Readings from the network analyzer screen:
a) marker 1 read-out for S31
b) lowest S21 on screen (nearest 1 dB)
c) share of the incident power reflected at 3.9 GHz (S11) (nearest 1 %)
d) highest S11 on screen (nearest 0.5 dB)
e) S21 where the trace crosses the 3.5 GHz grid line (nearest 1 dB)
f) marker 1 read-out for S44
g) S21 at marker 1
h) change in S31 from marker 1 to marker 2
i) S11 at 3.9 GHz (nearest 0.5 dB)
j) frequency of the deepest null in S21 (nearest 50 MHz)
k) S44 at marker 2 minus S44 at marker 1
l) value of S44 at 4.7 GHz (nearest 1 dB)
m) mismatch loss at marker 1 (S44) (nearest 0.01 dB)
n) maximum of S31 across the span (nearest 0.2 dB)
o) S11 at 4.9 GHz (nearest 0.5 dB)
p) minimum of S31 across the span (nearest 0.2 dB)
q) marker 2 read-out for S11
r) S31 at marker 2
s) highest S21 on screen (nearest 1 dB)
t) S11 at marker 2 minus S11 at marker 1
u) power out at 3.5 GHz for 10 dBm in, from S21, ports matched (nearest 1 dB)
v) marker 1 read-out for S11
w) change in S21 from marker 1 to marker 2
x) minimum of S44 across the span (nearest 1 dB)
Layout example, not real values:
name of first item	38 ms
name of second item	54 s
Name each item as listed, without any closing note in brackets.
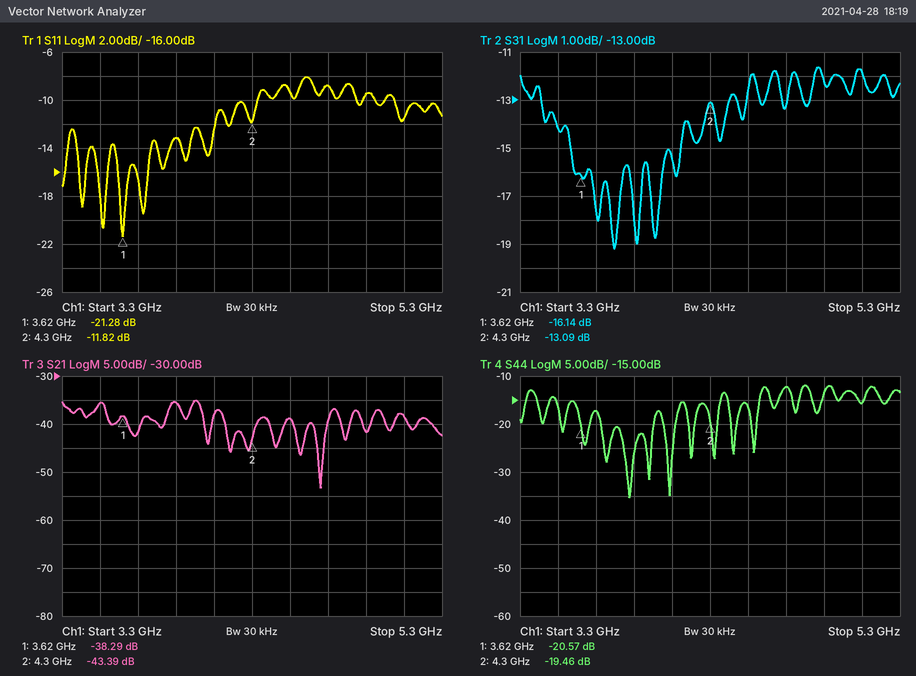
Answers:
marker 1 read-out for S31	-16.14 dB
lowest S21 on screen	-53 dB
share of the incident power reflected at 3.9 GHz (S11)	5 %
highest S11 on screen	-8.0 dB
S21 where the trace crosses the 3.5 GHz grid line	-36 dB
marker 1 read-out for S44	-20.57 dB
S21 at marker 1	-38.29 dB
change in S31 from marker 1 to marker 2	3.05 dB
S11 at 3.9 GHz	-13.0 dB
frequency of the deepest null in S21	4.65 GHz
S44 at marker 2 minus S44 at marker 1	1.11 dB
value of S44 at 4.7 GHz	-12 dB
mismatch loss at marker 1 (S44)	0.04 dB
maximum of S31 across the span	-11.6 dB
S11 at 4.9 GHz	-9.5 dB
minimum of S31 across the span	-19.2 dB
marker 2 read-out for S11	-11.82 dB
S31 at marker 2	-13.09 dB
highest S21 on screen	-35 dB
S11 at marker 2 minus S11 at marker 1	9.46 dB
power out at 3.5 GHz for 10 dBm in, from S21, ports matched	-26 dBm
marker 1 read-out for S11	-21.28 dB
change in S21 from marker 1 to marker 2	-5.10 dB
minimum of S44 across the span	-35 dB
